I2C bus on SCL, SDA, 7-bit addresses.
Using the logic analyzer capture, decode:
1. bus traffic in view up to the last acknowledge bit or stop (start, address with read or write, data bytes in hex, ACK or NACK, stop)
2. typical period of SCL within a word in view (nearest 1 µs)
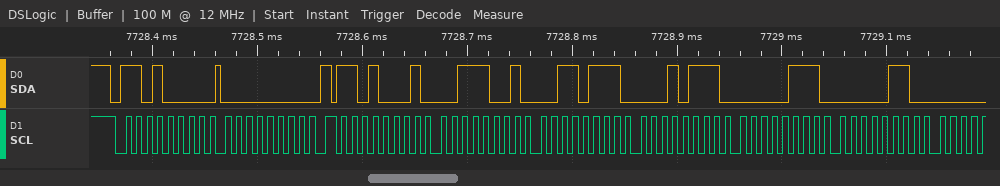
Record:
start, address 68 write ACK, 00 ACK, repeated start, address 68 read ACK, 39 ACK, 37 ACK, 17 ACK, 07 ACK, 06 ACK
10 µs
